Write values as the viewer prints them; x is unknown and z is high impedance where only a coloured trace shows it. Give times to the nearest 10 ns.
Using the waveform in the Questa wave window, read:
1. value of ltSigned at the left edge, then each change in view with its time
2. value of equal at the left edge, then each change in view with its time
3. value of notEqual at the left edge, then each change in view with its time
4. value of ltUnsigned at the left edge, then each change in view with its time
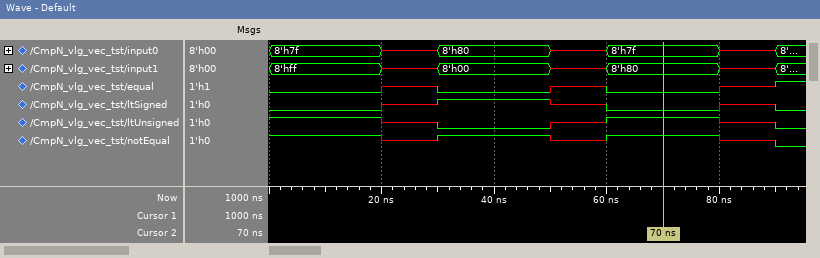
0, x at 20 ns, 1 at 30 ns, x at 50 ns, 0 at 60 ns, x at 80 ns, 0 at 90 ns
0, x at 20 ns, 0 at 30 ns, x at 50 ns, 0 at 60 ns, x at 80 ns, 1 at 90 ns
1, x at 20 ns, 1 at 30 ns, x at 50 ns, 1 at 60 ns, x at 80 ns, 0 at 90 ns
1, x at 20 ns, 0 at 30 ns, x at 50 ns, 1 at 60 ns, x at 80 ns, 0 at 90 ns
